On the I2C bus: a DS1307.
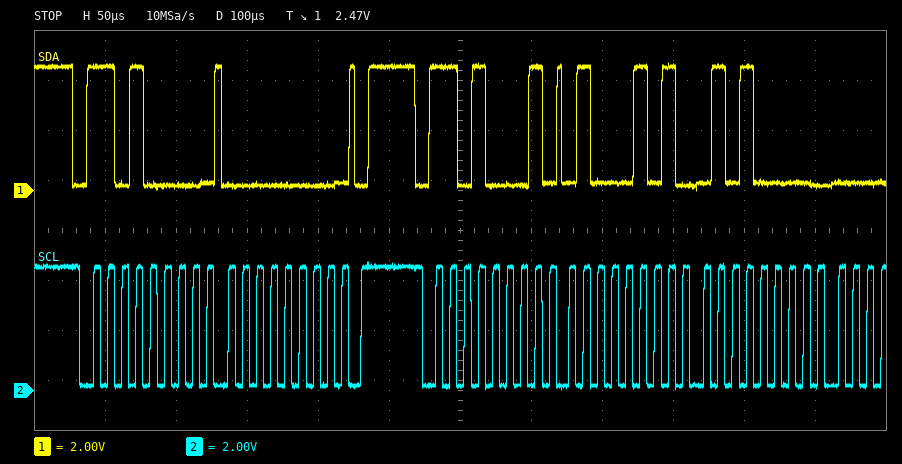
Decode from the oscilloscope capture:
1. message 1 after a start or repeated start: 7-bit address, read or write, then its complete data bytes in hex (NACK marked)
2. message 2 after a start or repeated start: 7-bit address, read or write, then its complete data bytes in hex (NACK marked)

0x68 write: 00
0x68 read: 45 50
